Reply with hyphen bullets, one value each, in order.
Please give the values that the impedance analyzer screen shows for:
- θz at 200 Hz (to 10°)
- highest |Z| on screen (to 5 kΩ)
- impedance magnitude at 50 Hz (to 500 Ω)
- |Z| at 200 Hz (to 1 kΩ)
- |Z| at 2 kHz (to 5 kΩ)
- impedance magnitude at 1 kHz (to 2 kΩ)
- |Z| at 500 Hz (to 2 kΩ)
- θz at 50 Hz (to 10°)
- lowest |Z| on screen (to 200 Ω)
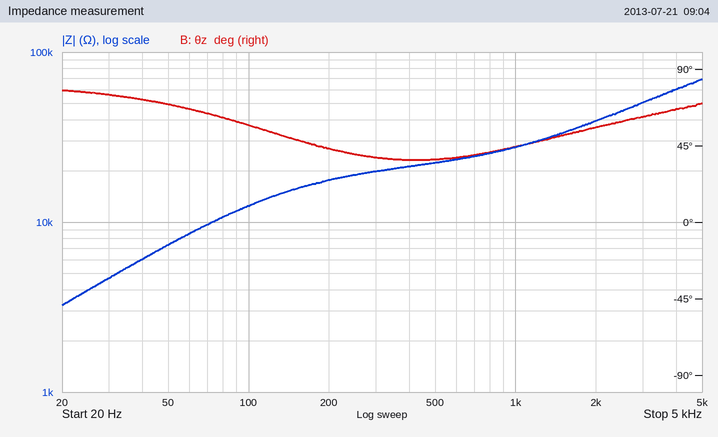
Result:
- 40°
- 70 kΩ
- 7.5 kΩ
- 18 kΩ
- 40 kΩ
- 28 kΩ
- 22 kΩ
- 70°
- 3.2 kΩ
